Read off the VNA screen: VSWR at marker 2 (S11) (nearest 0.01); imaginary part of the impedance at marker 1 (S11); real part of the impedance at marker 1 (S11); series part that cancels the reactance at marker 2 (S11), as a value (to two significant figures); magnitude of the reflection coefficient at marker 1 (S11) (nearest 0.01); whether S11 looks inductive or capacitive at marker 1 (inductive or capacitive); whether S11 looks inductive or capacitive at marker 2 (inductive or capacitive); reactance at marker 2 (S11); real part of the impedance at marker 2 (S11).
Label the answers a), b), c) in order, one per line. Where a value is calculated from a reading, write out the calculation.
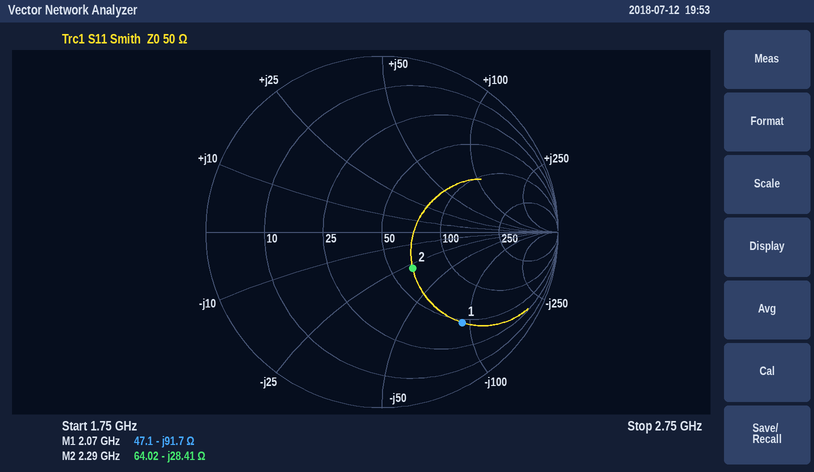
a) 1.74
b) -91.7 Ω
c) 47.1 Ω
d) L = 28.41 Ω/(2π × 2.29 GHz) ≈ 2.0 nH
e) 0.69
f) capacitive
g) capacitive
h) -28.41 Ω
i) 64.02 Ω
